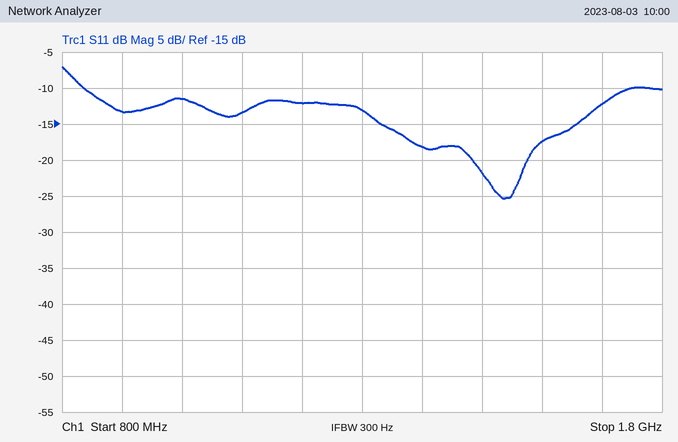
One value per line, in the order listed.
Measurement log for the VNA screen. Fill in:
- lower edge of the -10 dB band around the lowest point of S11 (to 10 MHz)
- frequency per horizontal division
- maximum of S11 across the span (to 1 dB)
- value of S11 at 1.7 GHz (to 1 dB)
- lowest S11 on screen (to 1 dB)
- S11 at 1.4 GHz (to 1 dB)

840 MHz
100 MHz
-7 dB
-12 dB
-25 dB
-18 dB
